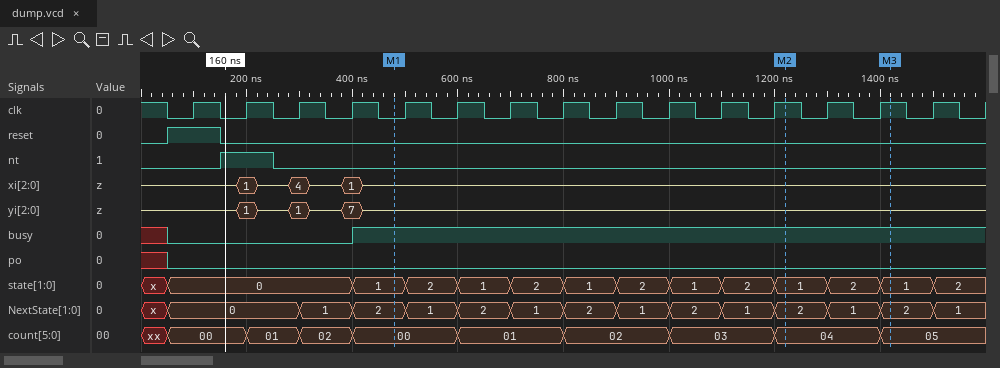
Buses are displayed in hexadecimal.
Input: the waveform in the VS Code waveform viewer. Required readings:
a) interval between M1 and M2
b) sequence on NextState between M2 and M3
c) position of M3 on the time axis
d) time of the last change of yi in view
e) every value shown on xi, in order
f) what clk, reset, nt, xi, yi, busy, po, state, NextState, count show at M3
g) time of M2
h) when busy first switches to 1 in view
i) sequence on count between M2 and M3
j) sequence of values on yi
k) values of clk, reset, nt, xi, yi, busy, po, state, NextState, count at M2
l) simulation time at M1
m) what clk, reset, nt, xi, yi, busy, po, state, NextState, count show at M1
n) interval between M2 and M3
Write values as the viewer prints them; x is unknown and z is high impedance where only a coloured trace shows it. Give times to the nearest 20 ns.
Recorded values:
740 ns
2, 1, 2
1420 ns
420 ns
z, 1, z, 4, z, 1, z
clk=1, reset=0, nt=0, xi=z, yi=z, busy=1, po=0, state=1, NextState=2, count=05
1220 ns
400 ns
04, 05
z, 1, z, 1, z, 7, z
clk=1, reset=0, nt=0, xi=z, yi=z, busy=1, po=0, state=1, NextState=2, count=04
480 ns
clk=0, reset=0, nt=0, xi=z, yi=z, busy=1, po=0, state=1, NextState=2, count=00
200 ns
